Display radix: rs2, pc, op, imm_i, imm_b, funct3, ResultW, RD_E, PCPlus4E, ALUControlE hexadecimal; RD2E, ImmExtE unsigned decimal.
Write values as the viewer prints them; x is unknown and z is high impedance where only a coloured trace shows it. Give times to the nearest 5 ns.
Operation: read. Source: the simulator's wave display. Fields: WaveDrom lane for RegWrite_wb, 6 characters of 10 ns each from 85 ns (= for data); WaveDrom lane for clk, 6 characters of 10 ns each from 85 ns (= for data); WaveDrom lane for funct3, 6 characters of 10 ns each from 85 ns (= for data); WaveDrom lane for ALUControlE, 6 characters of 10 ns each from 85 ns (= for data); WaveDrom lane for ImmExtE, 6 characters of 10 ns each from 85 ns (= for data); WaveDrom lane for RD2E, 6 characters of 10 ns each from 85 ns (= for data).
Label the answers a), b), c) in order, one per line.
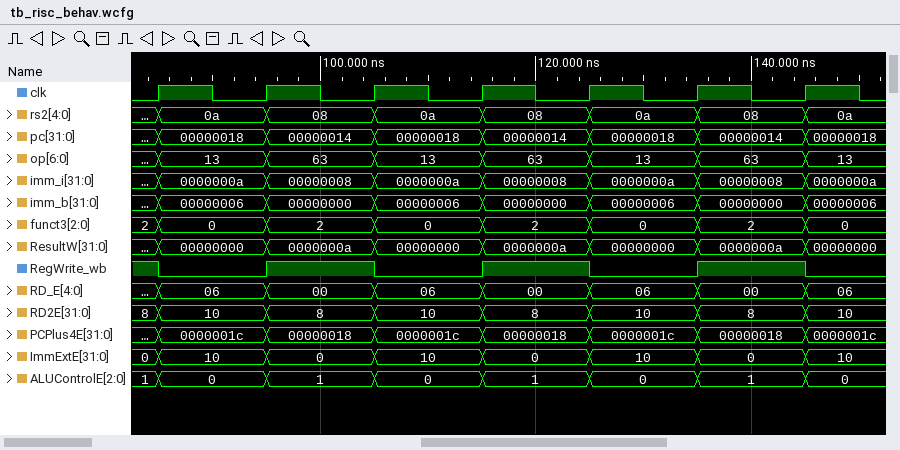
a) {name: 'RegWrite_wb', wave: '010101'}
b) {name: 'clk', wave: 'p.....'}
c) {name: 'funct3', wave: '======', data: '0 2 0 2 0 2'}
d) {name: 'ALUControlE', wave: '======', data: '0 1 0 1 0 1'}
e) {name: 'ImmExtE', wave: '======', data: '10 0 10 0 10 0'}
f) {name: 'RD2E', wave: '======', data: '10 8 10 8 10 8'}
